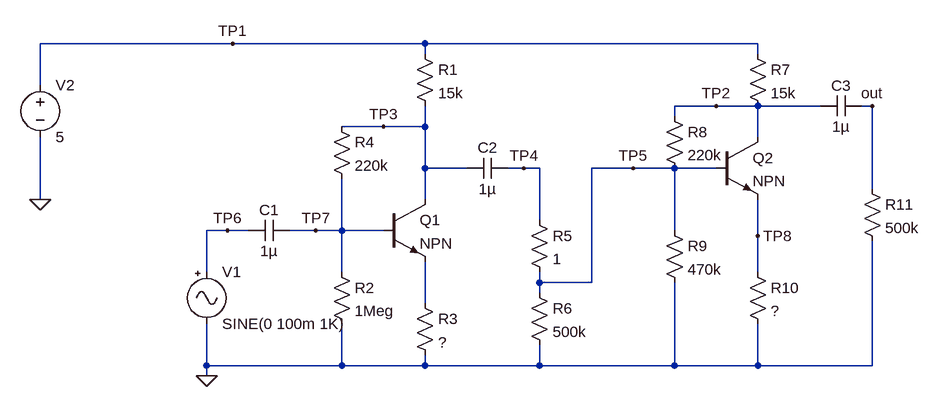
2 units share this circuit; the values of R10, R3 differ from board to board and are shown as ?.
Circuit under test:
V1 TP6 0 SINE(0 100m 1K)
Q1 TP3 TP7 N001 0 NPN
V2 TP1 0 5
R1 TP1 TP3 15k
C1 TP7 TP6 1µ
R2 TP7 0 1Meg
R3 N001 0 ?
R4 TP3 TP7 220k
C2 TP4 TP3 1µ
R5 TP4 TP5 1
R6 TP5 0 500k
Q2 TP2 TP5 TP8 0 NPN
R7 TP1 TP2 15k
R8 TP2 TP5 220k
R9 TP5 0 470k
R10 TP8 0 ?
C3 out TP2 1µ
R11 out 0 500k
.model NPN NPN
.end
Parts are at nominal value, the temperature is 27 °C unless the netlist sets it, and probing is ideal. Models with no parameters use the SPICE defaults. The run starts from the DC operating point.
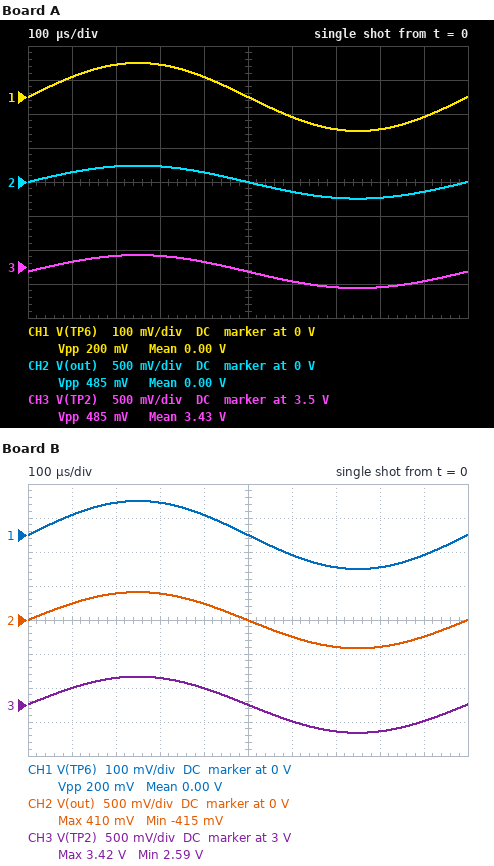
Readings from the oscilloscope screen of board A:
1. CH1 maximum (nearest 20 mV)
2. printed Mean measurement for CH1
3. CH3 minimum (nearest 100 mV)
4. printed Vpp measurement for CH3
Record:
100 mV
0.00 V
3.2 V
485 mV
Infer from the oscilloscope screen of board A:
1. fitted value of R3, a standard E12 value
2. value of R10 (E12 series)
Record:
5.6 kΩ
10 kΩ
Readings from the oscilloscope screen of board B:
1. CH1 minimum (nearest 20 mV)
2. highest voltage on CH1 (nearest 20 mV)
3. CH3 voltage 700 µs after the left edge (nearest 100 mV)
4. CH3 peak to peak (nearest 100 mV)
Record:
-100 mV
100 mV
2.6 V
800 mV
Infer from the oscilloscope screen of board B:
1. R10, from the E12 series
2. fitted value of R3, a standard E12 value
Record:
5.6 kΩ
5.6 kΩ
